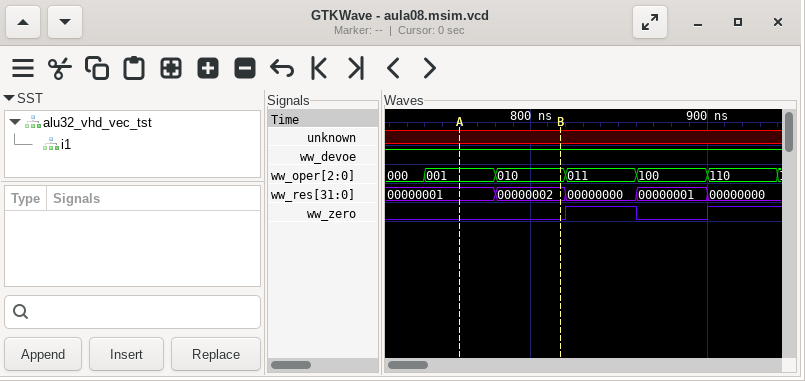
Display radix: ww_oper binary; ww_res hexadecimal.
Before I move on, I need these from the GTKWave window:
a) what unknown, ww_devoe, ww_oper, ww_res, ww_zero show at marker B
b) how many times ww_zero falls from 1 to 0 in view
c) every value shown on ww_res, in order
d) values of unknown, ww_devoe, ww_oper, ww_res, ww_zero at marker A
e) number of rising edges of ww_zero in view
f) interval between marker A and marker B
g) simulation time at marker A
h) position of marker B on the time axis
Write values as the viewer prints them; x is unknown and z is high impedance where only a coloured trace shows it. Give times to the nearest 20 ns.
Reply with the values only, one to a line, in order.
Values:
unknown=x, ww_devoe=1, ww_oper=010, ww_res=00000002, ww_zero=0
1
00000001, 00000002, 00000000, 00000001, 00000000
unknown=x, ww_devoe=1, ww_oper=001, ww_res=00000001, ww_zero=0
2
60 ns
760 ns
820 ns
